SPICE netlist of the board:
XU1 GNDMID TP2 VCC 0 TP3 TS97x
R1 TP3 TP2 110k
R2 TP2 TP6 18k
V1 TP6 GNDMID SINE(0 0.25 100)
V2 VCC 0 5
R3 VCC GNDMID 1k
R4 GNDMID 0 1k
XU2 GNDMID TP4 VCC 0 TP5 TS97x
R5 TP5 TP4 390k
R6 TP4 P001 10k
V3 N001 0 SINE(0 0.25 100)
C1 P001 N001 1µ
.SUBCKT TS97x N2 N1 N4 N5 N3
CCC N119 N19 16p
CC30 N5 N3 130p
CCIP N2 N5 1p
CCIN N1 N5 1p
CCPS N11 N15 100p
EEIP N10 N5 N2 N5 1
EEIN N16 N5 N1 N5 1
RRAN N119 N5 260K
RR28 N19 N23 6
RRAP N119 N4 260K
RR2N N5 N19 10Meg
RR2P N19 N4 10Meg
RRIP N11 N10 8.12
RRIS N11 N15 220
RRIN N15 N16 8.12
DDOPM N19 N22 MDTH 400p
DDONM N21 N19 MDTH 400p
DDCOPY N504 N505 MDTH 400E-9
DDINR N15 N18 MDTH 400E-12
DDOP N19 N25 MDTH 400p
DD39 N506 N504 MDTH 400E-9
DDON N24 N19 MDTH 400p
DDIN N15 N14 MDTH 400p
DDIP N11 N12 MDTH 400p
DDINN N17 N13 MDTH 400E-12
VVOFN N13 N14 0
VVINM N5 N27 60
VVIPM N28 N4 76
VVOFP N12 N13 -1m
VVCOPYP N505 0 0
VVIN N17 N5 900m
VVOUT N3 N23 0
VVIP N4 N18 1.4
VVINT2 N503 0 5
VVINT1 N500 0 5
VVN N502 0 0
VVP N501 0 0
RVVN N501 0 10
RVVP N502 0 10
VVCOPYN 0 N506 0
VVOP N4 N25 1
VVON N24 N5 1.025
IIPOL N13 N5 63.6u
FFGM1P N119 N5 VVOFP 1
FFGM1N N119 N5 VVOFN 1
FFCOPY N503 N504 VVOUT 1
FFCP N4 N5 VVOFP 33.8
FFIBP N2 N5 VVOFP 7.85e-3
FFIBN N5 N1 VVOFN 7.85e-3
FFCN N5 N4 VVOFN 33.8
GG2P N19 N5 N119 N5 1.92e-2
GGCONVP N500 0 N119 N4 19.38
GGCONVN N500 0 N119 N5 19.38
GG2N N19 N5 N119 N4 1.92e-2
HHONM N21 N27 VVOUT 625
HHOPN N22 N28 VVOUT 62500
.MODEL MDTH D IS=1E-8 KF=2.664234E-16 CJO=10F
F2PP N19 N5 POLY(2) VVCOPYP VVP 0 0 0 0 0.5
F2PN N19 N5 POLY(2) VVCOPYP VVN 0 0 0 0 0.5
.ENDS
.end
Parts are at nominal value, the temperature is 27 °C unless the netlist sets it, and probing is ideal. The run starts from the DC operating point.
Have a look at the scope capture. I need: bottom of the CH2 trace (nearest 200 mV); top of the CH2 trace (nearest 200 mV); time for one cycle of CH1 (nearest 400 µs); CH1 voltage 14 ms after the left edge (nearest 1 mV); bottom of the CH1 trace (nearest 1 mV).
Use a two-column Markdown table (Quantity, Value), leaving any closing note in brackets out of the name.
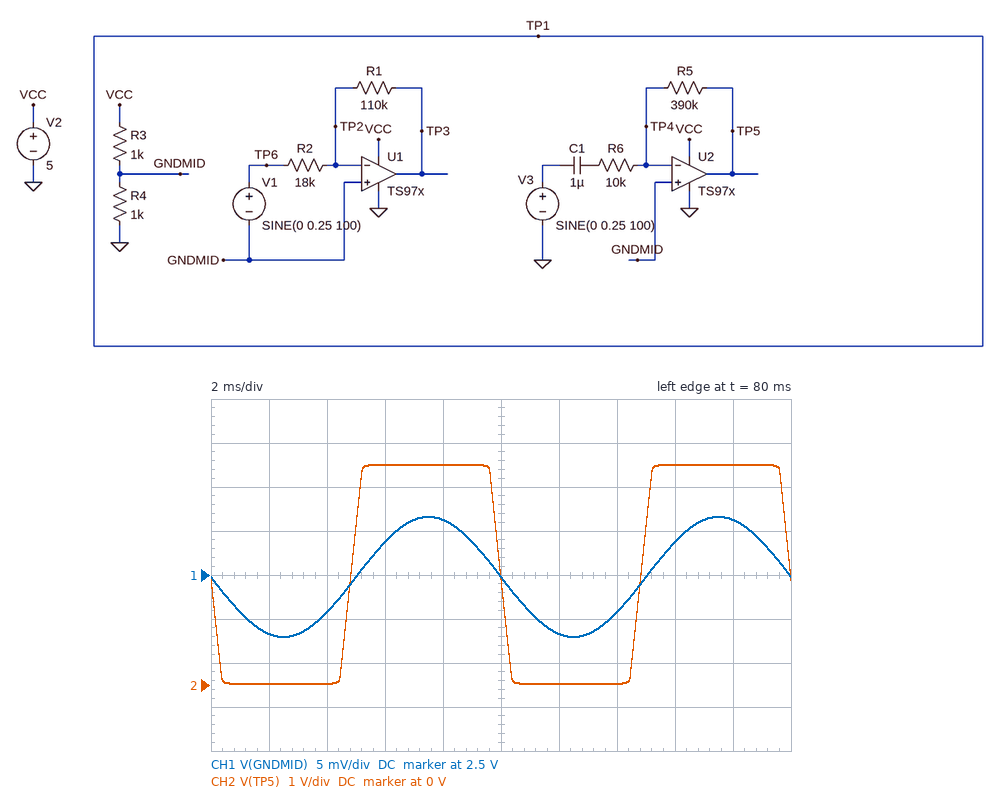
| Quantity | Value |
|---|---|
| bottom of the CH2 trace | 0 V |
| top of the CH2 trace | 5.0 V |
| time for one cycle of CH1 | 10.0 ms |
| CH1 voltage 14 ms after the left edge | 2.496 V |
| bottom of the CH1 trace | 2.493 V |
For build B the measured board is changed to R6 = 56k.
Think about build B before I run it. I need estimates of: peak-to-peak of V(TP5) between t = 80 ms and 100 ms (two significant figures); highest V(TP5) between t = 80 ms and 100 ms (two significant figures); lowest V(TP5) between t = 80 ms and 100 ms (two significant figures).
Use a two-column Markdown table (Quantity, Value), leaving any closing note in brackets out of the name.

| Quantity | Value |
|---|---|
| peak-to-peak of V(TP5) between t = 80 ms and 100 ms | 3.6 V |
| highest V(TP5) between t = 80 ms and 100 ms | 4.4 V |
| lowest V(TP5) between t = 80 ms and 100 ms | 810 mV |
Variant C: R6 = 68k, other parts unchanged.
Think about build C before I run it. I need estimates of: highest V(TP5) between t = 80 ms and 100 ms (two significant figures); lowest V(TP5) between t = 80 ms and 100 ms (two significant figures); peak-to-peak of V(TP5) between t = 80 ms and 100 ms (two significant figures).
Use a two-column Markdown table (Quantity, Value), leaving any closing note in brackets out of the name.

| Quantity | Value |
|---|---|
| highest V(TP5) between t = 80 ms and 100 ms | 4.1 V |
| lowest V(TP5) between t = 80 ms and 100 ms | 1.1 V |
| peak-to-peak of V(TP5) between t = 80 ms and 100 ms | 3.0 V |
